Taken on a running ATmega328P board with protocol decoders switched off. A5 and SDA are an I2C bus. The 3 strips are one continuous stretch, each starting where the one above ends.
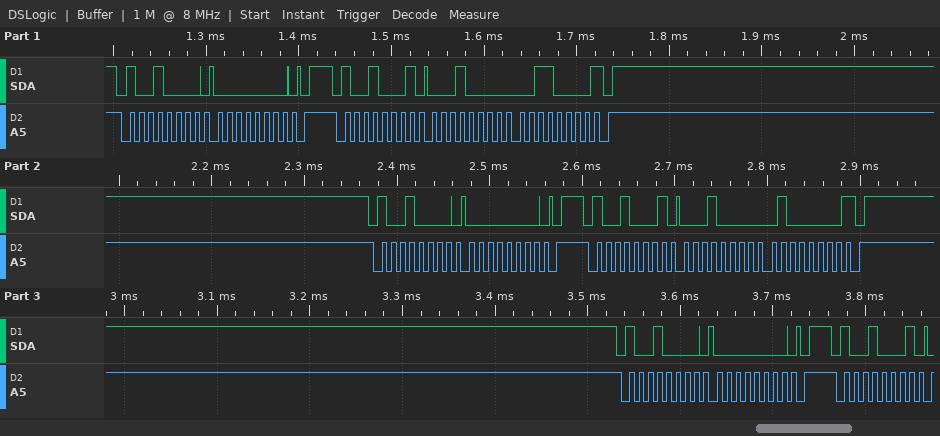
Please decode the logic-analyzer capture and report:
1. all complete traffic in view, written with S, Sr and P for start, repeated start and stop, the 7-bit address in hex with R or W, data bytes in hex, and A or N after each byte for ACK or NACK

S 48W A 00 A P S 48R A 10 A 30 N P S 48W A 00 A P S 48R A 10 A 40 N P S 48W A 00 A P S 48R A
